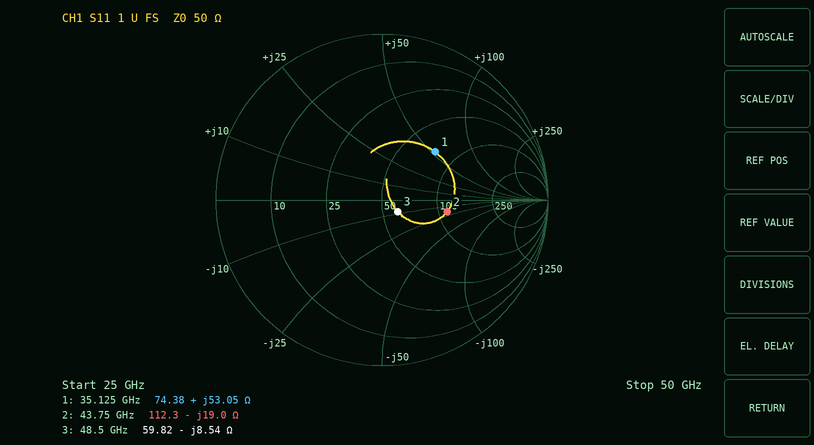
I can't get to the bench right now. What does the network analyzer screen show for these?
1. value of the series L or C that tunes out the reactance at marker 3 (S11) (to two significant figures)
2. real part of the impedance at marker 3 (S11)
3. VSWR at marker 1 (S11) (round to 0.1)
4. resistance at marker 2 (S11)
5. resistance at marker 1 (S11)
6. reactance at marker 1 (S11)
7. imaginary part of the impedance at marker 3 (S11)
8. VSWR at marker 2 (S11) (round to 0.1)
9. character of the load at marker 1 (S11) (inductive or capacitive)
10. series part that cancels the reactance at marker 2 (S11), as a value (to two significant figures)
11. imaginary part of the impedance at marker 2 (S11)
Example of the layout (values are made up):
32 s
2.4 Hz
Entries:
28 pH
59.82 Ω
2.5
112.3 Ω
74.38 Ω
+53.05 Ω
-8.54 Ω
2.3
inductive
69 pH
-19.0 Ω
